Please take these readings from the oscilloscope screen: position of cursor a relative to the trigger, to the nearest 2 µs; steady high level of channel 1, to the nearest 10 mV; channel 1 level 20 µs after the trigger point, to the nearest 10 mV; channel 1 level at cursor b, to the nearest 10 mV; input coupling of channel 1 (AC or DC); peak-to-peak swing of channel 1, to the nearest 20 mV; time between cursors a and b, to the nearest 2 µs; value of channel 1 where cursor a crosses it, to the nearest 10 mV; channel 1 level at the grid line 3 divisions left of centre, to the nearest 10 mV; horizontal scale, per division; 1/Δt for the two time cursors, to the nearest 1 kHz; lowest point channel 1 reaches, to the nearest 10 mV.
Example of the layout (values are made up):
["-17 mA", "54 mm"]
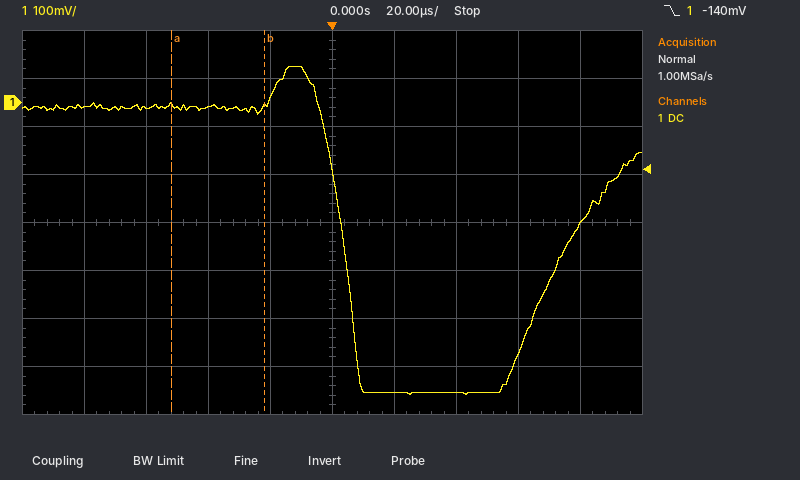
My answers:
["-52 µs", "-10 mV", "-600 mV", "-10 mV", "DC", "680 mV", "30 µs", "-10 mV", "-10 mV", "20 µs", "33 kHz", "-610 mV"]
